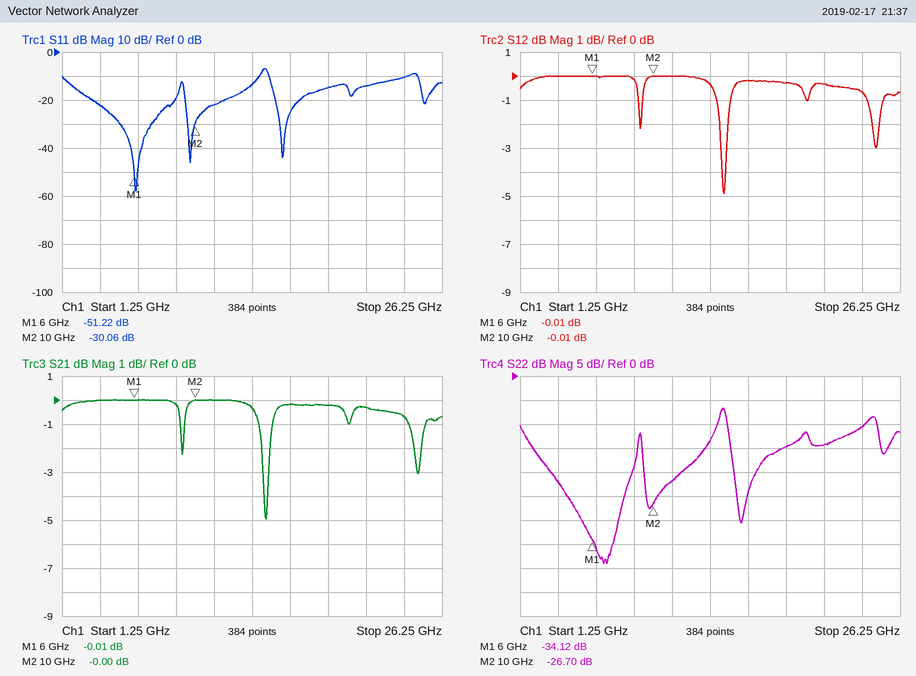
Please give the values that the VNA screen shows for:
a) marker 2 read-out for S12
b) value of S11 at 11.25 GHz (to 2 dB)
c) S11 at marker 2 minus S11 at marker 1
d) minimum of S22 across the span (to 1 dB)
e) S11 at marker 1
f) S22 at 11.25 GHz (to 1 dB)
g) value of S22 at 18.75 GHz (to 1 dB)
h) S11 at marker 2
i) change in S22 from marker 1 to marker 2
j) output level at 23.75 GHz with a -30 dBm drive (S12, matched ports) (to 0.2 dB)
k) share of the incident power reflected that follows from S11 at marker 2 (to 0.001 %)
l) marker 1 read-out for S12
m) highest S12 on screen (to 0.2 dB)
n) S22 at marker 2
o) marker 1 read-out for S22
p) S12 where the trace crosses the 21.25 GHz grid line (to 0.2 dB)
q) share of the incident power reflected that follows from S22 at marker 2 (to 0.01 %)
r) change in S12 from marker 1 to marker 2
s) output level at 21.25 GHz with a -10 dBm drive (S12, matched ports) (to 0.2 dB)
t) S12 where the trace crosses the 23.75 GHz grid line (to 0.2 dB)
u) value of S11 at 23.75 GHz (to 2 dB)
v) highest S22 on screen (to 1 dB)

-0.01 dB
-22 dB
21.16 dB
-39 dB
-51.22 dB
-22 dB
-15 dB
-30.06 dB
7.42 dB
-30.6 dBm
0.099 %
-0.01 dB
0.0 dB
-26.70 dB
-34.12 dB
-0.4 dB
0.21 %
0.00 dB
-10.4 dBm
-0.6 dB
-10 dB
-7 dB
